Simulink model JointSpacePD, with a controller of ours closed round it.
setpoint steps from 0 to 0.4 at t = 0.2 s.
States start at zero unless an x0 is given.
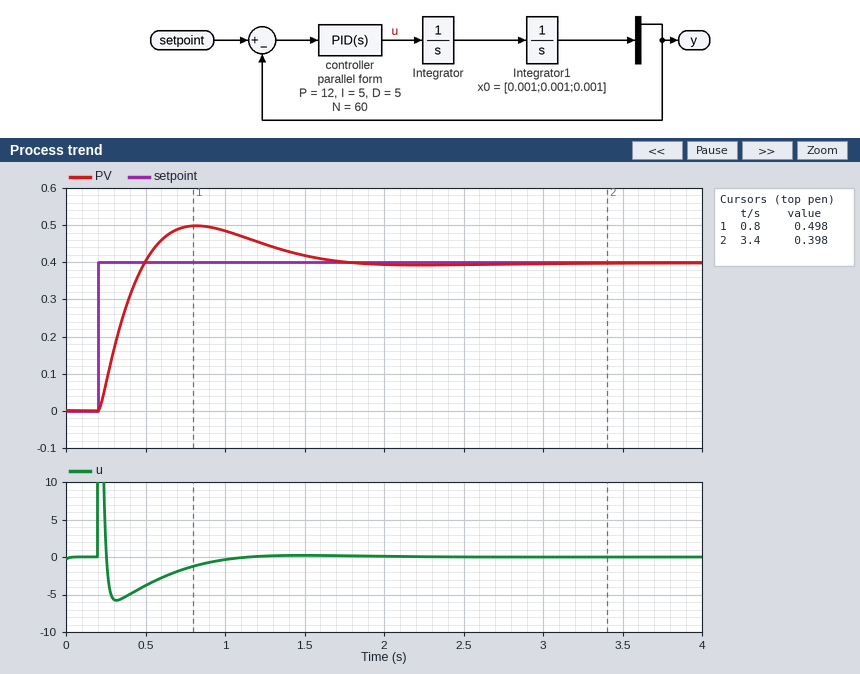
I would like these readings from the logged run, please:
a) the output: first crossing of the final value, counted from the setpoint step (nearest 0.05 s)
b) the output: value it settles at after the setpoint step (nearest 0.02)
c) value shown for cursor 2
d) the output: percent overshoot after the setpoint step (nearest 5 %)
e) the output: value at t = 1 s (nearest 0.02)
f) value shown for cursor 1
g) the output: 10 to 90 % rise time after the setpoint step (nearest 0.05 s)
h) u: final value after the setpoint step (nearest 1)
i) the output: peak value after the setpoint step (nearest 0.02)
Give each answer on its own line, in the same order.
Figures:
0.30 s
0.40
0.398
25 %
0.48
0.498
0.20 s
0
0.50
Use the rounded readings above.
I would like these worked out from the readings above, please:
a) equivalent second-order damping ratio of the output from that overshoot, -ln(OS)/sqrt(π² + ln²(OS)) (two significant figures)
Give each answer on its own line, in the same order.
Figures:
0.40
